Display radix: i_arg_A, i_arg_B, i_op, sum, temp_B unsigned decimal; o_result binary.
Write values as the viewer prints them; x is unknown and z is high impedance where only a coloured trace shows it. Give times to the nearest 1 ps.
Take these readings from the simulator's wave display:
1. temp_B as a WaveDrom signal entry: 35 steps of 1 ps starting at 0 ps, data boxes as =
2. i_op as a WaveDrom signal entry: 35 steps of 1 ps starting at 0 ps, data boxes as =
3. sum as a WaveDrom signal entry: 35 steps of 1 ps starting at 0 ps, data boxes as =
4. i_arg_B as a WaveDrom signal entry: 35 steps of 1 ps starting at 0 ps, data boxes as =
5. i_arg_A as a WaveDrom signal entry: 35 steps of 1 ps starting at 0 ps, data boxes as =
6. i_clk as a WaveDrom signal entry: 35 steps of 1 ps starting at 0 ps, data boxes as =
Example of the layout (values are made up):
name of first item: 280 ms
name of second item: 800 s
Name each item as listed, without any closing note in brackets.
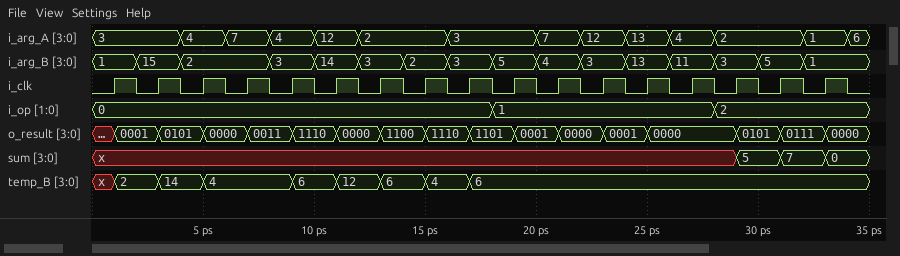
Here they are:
temp_B as a WaveDrom signal entry: 35 steps of 1 ps starting at 0 ps, data boxes as =: {name: 'temp_B', wave: 'x=.=.=...=.=.=.=.=.................', data: '2 14 4 6 12 6 4 6'}
i_op as a WaveDrom signal entry: 35 steps of 1 ps starting at 0 ps, data boxes as =: {name: 'i_op', wave: '=.................=.........=......', data: '0 1 2'}
sum as a WaveDrom signal entry: 35 steps of 1 ps starting at 0 ps, data boxes as =: {name: 'sum', wave: 'x............................=.=.=.', data: '5 7 0'}
i_arg_B as a WaveDrom signal entry: 35 steps of 1 ps starting at 0 ps, data boxes as =: {name: 'i_arg_B', wave: '=.=.=...=.=.=.=.=.=.=.=.=.=.=.=.=..', data: '1 15 2 3 14 3 2 3 5 4 3 13 11 3 5 1'}
i_arg_A as a WaveDrom signal entry: 35 steps of 1 ps starting at 0 ps, data boxes as =: {name: 'i_arg_A', wave: '=...=.=.=.=.=...=...=.=.=.=.=...=.=', data: '3 4 7 4 12 2 3 7 12 13 4 2 1 6'}
i_clk as a WaveDrom signal entry: 35 steps of 1 ps starting at 0 ps, data boxes as =: {name: 'i_clk', wave: '01010101010101010101010101010101010'}
